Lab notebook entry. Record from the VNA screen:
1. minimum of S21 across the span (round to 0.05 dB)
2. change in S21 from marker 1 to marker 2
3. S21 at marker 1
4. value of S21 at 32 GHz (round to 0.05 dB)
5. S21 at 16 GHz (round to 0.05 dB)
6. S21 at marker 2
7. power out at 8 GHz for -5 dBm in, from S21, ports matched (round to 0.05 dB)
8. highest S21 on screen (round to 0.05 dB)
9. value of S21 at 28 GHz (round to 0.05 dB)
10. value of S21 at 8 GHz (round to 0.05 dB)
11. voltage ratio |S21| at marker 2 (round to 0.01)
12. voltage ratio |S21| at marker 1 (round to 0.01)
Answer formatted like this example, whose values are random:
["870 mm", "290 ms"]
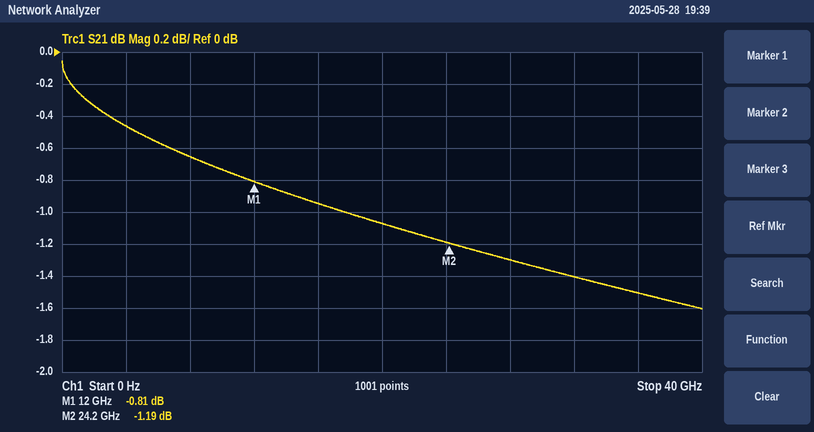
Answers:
["-1.60 dB", "-0.38 dB", "-0.81 dB", "-1.40 dB", "-0.95 dB", "-1.19 dB", "-5.65 dBm", "-0.05 dB", "-1.30 dB", "-0.65 dB", "0.87", "0.91"]
